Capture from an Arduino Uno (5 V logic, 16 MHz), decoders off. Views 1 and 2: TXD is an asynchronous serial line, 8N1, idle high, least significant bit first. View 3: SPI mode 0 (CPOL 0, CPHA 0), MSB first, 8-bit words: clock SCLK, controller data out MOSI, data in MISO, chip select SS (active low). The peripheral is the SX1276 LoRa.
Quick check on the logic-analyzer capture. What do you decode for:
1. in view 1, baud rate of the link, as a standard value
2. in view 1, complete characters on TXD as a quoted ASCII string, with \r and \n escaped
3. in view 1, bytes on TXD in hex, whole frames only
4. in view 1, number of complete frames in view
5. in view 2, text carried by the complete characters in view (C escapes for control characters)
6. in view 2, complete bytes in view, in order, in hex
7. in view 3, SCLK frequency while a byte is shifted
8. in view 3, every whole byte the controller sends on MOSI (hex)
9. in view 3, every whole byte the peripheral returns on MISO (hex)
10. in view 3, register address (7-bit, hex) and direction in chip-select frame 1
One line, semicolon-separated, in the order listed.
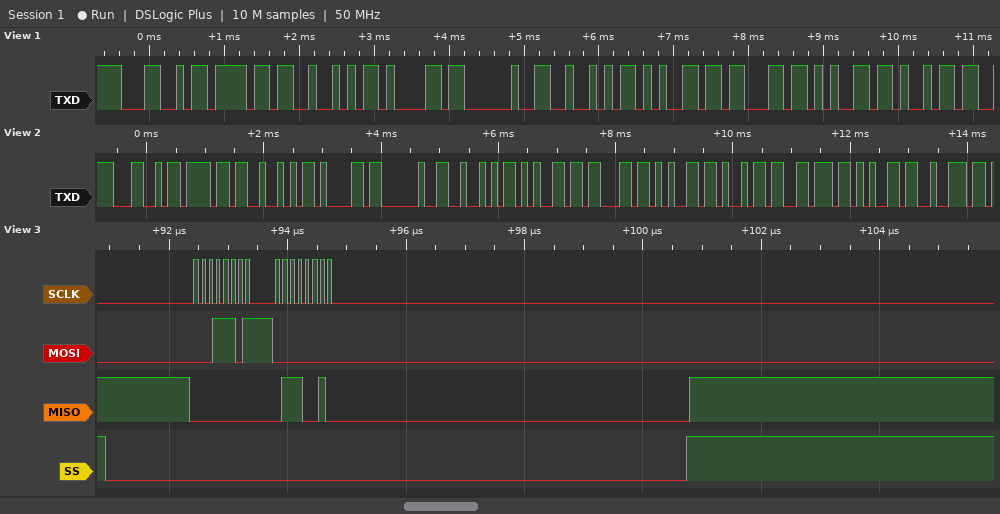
9600 baud; "LoRa Recei"; 4C 6F 52 61 20 52 65 63 65 69; 10; "LoRa Receiver"; 0x4C 0x6F 0x52 0x61 0x20 0x52 0x65 0x63 0x65 0x69 0x76 0x65 0x72; 8 MHz; 1D 00; 00 72; 0x1D read
